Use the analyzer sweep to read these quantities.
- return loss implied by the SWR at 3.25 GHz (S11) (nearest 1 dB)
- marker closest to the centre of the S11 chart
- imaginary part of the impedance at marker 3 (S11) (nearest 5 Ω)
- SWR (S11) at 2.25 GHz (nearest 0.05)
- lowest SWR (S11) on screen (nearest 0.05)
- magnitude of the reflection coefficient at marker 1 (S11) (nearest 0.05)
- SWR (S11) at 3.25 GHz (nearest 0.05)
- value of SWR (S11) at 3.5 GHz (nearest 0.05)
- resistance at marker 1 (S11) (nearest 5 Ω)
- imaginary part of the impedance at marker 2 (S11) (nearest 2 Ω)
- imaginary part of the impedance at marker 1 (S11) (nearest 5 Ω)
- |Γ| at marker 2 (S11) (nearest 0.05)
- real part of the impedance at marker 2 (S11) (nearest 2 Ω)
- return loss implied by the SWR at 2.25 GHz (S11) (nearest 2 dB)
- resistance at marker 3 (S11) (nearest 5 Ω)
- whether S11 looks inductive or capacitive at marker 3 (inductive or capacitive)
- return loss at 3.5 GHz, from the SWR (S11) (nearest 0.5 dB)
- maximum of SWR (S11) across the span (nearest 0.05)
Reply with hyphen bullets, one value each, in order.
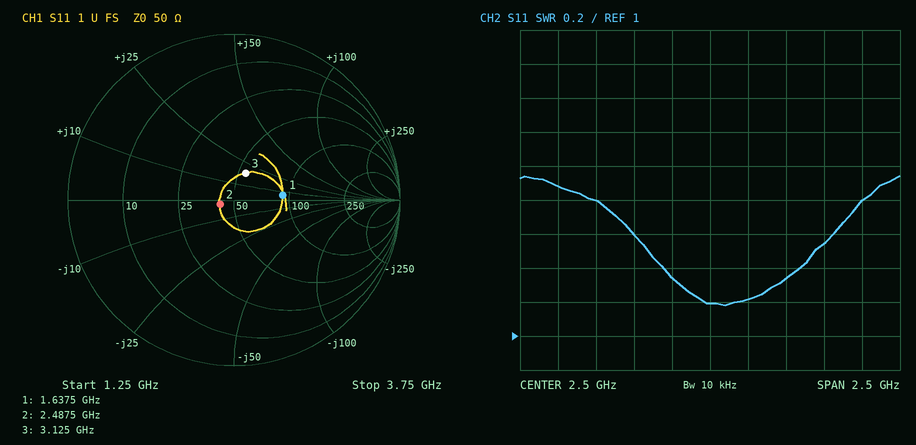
- 13 dB
- marker 2
- +20 Ω
- 1.35
- 1.20
- 0.30
- 1.55
- 1.80
- 90 Ω
- -2 Ω
- +5 Ω
- 0.10
- 42 Ω
- 16 dB
- 55 Ω
- inductive
- 11.0 dB
- 1.95
